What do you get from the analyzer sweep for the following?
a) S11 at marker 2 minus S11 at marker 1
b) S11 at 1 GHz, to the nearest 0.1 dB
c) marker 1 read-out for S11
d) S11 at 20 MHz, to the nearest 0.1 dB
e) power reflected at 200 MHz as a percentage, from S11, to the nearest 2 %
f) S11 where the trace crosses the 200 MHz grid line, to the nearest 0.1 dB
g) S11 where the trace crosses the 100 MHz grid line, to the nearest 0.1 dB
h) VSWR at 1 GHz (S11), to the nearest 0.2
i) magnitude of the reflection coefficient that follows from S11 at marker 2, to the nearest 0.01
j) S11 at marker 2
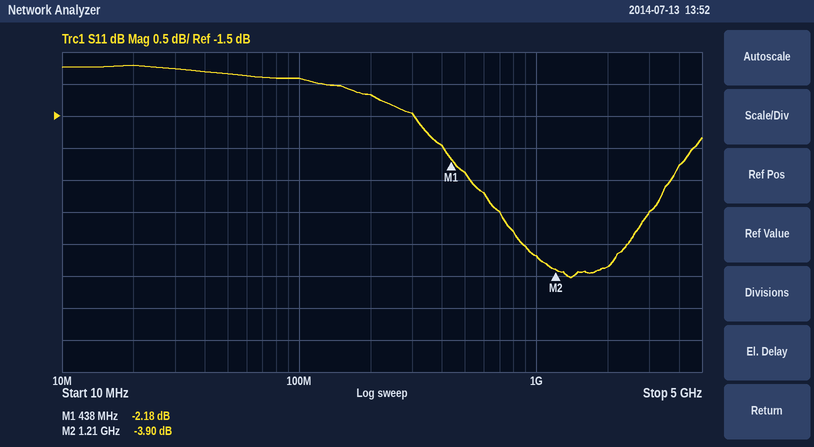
-1.72 dB
-3.7 dB
-2.18 dB
-0.7 dB
76 %
-1.2 dB
-0.9 dB
4.8
0.64
-3.90 dB
